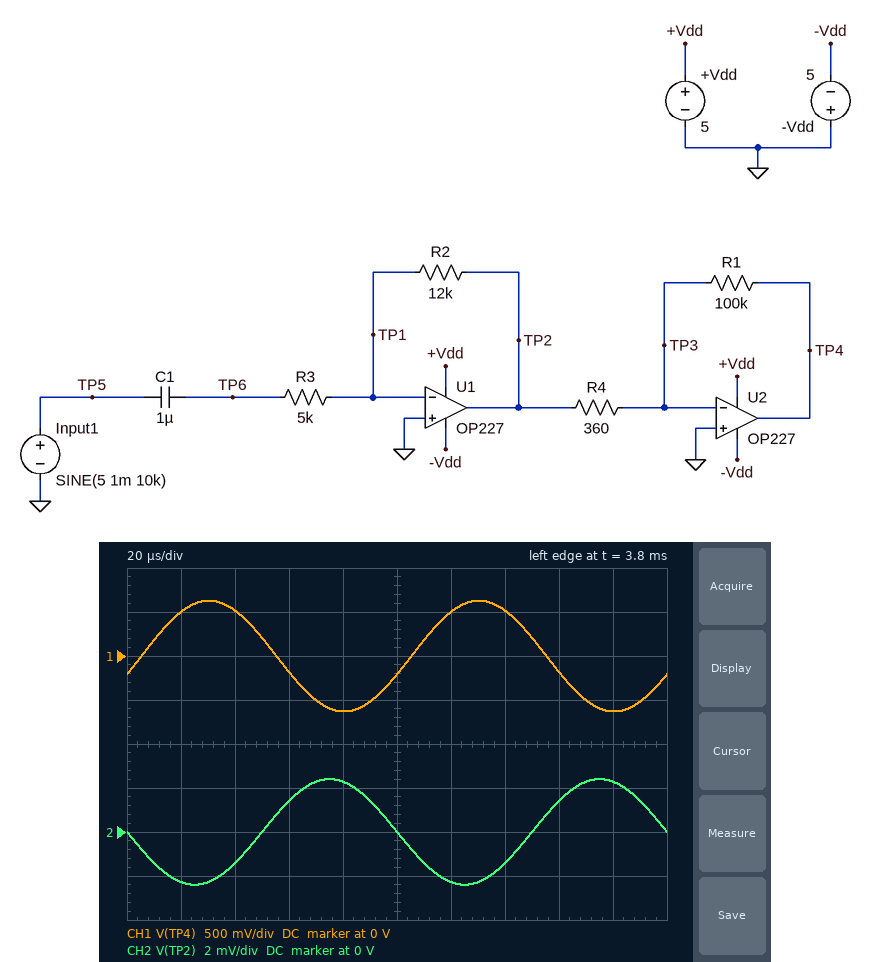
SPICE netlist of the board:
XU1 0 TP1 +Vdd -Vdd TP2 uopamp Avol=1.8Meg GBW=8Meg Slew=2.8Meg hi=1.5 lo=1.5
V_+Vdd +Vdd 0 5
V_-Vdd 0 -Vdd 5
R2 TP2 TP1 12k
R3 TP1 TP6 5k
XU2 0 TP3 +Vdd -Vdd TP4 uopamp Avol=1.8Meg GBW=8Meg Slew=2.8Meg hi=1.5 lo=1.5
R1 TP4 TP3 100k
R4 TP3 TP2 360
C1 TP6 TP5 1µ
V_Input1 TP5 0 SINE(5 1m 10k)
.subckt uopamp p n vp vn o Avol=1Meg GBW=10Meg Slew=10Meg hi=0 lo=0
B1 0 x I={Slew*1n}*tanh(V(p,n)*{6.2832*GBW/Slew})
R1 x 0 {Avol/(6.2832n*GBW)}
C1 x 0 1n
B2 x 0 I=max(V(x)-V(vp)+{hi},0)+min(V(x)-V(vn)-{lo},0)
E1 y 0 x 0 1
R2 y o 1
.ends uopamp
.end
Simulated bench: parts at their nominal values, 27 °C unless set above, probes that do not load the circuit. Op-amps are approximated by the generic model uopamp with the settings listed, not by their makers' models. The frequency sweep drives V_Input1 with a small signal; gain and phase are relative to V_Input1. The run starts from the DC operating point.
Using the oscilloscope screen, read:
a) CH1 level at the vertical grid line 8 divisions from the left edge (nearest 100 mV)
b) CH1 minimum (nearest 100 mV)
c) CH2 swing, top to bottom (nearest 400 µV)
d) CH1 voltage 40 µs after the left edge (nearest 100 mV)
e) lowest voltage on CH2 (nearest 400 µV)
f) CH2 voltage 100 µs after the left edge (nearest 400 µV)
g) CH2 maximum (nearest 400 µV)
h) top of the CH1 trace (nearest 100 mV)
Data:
-200 mV
-600 mV
4.8 mV
500 mV
-2.4 mV
0 V
2.4 mV
600 mV
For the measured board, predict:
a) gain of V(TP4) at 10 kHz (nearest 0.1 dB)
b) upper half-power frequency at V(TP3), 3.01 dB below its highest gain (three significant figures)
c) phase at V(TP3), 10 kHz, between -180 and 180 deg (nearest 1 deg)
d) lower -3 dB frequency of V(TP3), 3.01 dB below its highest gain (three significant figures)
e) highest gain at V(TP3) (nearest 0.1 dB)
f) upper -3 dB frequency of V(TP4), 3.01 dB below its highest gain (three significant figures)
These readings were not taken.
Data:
56.0 dB
2.41 MHz
-109 deg
28.0 kHz
7.5 dB
28.8 kHz
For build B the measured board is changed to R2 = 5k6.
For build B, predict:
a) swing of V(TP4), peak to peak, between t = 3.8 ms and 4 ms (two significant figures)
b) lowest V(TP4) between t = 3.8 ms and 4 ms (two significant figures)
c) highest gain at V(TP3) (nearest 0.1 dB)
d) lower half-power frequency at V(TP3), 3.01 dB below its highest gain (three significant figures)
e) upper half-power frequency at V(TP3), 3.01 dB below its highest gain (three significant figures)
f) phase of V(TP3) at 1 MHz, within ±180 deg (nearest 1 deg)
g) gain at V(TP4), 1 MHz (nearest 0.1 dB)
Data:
590 mV
-290 mV
0.9 dB
28.3 kHz
3.83 MHz
167 deg
18.7 dB
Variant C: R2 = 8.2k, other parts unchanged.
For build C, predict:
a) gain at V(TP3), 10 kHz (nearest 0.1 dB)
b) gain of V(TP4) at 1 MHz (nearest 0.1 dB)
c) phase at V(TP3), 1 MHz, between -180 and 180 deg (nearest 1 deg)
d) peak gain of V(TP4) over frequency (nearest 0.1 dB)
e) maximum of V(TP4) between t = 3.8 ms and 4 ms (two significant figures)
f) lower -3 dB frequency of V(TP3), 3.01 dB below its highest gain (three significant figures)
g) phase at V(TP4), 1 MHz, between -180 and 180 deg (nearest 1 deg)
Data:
-5.4 dB
21.9 dB
163 deg
53.2 dB
430 mV
28.2 kHz
-107 deg
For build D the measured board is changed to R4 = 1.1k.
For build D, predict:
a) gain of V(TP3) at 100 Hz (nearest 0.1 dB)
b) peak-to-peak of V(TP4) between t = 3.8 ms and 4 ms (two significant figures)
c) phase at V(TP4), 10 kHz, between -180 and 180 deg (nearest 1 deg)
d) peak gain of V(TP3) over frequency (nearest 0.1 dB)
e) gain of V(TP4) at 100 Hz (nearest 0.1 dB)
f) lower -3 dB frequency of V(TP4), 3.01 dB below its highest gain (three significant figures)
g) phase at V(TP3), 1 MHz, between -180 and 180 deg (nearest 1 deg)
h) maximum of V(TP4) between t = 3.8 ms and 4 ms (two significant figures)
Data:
-51.7 dB
430 mV
-7 deg
7.2 dB
46.4 dB
31.8 Hz
162 deg
220 mV
